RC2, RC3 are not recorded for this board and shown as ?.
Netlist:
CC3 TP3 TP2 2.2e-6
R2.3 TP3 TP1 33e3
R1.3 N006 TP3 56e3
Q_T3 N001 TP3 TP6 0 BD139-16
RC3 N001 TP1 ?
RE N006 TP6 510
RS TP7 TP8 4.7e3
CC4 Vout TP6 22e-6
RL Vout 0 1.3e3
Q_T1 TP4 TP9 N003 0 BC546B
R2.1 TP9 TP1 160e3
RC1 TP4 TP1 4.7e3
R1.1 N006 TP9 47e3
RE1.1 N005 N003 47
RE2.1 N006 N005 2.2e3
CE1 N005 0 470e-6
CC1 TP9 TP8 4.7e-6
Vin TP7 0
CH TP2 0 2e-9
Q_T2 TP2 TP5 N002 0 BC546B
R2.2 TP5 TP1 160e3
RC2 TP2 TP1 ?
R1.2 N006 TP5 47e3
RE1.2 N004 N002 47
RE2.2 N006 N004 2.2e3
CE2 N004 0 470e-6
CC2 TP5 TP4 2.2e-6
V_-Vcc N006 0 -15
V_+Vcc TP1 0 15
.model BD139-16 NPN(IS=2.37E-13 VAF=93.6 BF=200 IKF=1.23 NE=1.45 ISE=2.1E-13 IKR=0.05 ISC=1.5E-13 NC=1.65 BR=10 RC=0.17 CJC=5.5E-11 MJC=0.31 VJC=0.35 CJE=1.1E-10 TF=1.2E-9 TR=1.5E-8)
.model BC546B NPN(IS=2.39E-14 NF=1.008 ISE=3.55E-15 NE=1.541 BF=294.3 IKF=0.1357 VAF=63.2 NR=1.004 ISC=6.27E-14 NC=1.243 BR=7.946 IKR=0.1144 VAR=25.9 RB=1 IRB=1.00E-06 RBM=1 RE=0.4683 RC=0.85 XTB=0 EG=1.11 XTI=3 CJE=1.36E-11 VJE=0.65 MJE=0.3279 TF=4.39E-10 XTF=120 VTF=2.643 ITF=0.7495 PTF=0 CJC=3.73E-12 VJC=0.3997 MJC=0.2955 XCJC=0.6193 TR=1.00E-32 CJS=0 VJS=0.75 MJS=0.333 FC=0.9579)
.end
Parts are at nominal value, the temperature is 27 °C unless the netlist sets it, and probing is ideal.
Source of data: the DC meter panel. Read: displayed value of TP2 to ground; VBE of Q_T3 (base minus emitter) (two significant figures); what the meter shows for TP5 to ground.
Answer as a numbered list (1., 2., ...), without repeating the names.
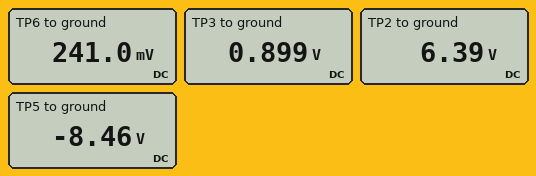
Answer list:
1. 6.39 V
2. 660 mV
3. -8.46 V
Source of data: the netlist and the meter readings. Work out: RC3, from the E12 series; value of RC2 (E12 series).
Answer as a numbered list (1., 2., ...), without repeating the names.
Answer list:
1. 68 Ω
2. 3.3 kΩ
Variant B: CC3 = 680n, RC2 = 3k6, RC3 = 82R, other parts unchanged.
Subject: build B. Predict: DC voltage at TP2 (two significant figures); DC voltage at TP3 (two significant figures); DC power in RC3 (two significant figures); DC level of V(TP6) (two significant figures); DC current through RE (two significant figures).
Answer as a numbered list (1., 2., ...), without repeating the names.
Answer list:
1. 5.6 V
2. 890 mV
3. 72 mW
4. 230 mV
5. 30 mA
